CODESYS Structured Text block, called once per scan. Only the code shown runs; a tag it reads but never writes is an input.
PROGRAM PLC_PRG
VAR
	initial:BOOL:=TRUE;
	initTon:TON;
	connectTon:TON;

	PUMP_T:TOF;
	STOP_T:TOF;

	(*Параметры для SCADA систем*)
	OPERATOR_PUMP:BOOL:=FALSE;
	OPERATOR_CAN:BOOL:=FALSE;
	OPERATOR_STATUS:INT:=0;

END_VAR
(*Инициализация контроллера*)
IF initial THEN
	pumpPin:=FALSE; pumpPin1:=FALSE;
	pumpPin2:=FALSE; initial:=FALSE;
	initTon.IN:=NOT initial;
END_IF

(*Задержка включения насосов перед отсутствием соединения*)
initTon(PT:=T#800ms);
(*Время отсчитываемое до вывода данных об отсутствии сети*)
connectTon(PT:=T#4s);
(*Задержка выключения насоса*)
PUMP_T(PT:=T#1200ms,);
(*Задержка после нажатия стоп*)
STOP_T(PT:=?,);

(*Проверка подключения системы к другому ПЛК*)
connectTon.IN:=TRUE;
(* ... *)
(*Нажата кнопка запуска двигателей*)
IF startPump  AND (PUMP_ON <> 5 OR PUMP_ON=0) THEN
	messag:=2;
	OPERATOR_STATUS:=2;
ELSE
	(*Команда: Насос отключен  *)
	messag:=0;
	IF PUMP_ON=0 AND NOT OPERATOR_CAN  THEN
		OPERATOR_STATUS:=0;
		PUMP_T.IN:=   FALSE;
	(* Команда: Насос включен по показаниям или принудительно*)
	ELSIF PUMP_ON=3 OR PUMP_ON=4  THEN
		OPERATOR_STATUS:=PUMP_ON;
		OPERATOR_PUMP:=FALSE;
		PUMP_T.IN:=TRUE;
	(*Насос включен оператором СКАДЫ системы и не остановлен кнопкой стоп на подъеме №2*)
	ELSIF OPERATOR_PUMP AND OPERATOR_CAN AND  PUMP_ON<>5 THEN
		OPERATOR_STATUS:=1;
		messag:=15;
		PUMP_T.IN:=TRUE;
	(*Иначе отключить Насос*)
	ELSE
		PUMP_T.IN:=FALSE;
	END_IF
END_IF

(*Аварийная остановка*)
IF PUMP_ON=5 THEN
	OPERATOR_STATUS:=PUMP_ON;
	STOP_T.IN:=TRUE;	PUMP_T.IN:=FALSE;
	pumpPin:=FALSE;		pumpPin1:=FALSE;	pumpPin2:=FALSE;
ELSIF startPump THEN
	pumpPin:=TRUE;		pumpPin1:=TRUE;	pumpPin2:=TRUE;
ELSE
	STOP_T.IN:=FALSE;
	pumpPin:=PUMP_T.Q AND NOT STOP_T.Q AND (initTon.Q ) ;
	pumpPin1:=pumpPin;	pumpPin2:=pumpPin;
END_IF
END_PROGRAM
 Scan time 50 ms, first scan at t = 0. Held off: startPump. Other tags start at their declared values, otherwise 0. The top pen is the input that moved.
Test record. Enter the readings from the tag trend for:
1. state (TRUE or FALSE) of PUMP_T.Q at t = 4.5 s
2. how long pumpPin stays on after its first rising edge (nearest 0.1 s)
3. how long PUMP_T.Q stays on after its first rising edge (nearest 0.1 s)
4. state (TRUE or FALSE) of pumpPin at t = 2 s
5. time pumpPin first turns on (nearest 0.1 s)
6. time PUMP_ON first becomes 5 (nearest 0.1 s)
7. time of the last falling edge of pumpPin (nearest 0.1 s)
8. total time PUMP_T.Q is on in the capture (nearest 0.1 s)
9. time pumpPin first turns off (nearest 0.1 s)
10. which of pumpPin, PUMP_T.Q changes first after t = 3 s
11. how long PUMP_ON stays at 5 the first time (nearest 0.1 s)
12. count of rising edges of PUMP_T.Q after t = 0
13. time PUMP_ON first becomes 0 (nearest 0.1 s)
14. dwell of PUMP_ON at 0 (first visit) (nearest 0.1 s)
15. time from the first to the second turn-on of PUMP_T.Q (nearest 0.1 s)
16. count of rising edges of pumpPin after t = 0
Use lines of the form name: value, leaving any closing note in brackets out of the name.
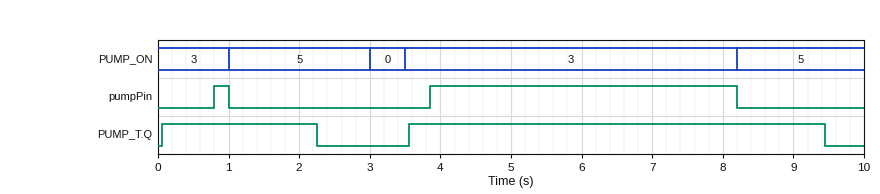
state (TRUE or FALSE) of PUMP_T.Q at t = 4.5 s: TRUE
how long pumpPin stays on after its first rising edge: 0.2 s
how long PUMP_T.Q stays on after its first rising edge: 2.2 s
state (TRUE or FALSE) of pumpPin at t = 2 s: FALSE
time pumpPin first turns on: 0.8 s
time PUMP_ON first becomes 5: 1.0 s
time of the last falling edge of pumpPin: 8.2 s
total time PUMP_T.Q is on in the capture: 8.1 s
time pumpPin first turns off: 1.0 s
which of pumpPin, PUMP_T.Q changes first after t = 3 s: PUMP_T.Q
how long PUMP_ON stays at 5 the first time: 2.0 s
count of rising edges of PUMP_T.Q after t = 0: 2
time PUMP_ON first becomes 0: 3.0 s
dwell of PUMP_ON at 0 (first visit): 0.5 s
time from the first to the second turn-on of PUMP_T.Q: 3.5 s
count of rising edges of pumpPin after t = 0: 2
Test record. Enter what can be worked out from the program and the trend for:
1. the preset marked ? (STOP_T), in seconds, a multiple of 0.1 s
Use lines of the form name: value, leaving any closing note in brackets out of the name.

the preset marked ? (STOP_T), in seconds, a multiple of 0.1 s: 0.8 s
